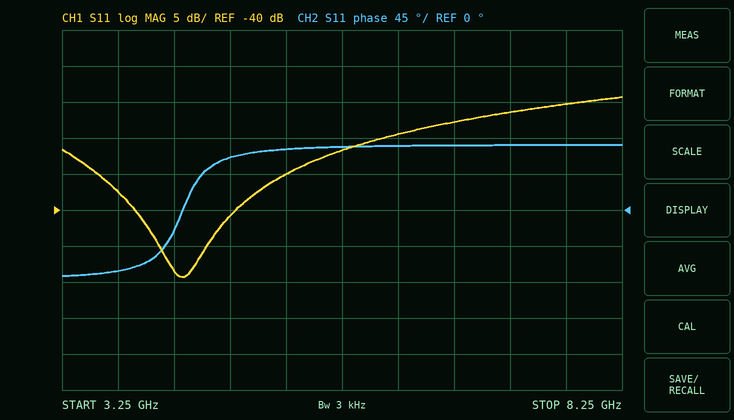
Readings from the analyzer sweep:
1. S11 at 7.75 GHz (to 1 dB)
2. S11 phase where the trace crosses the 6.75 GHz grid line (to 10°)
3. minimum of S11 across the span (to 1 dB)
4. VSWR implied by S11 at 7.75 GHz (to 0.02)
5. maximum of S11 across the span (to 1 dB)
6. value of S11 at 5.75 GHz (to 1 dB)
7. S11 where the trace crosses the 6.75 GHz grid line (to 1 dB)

-25 dB
80°
-49 dB
1.12
-24 dB
-32 dB
-28 dB
